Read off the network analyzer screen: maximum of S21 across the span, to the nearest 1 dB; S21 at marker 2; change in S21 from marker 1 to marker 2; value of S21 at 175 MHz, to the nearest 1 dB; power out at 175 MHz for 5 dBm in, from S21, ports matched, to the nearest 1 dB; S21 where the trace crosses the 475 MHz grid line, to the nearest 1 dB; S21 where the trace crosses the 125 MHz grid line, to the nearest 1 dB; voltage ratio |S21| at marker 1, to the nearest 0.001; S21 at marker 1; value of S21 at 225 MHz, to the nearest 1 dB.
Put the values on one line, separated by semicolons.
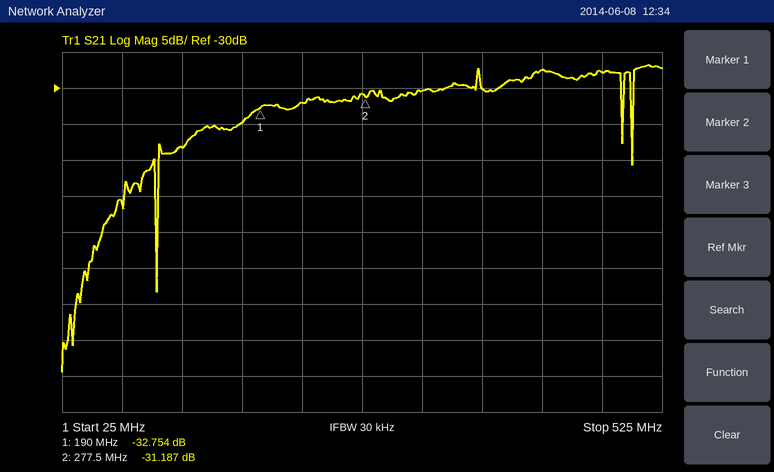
-27 dB; -31.187 dB; 1.567 dB; -35 dB; -30 dBm; -28 dB; -38 dB; 0.023; -32.754 dB; -32 dB
